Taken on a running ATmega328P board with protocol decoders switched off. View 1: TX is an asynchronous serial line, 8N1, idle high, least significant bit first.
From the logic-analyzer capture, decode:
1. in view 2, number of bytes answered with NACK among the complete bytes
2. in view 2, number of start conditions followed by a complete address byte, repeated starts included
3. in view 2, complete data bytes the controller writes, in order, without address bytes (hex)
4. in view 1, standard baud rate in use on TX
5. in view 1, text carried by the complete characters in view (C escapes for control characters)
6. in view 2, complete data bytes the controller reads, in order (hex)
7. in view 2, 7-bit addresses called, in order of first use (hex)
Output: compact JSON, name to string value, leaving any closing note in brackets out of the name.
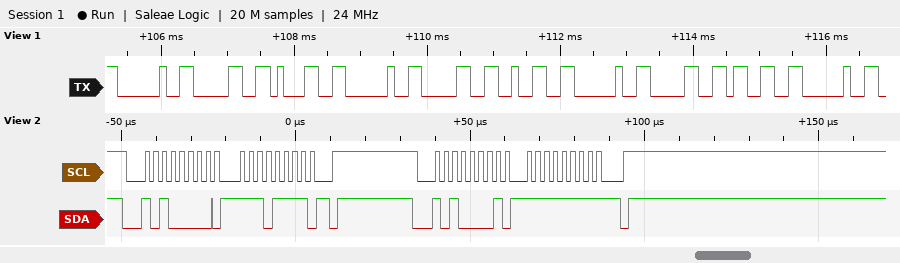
{"in view 2, number of bytes answered with NACK among the complete bytes": "1", "in view 2, number of start conditions followed by a complete address byte, repeated starts included": "2", "in view 2, complete data bytes the controller writes, in order, without address bytes": "EF", "in view 1, standard baud rate in use on TX": "9600 baud", "in view 1, text carried by the complete characters in view": "\" 01 02 03 \"", "in view 2, complete data bytes the controller reads, in order": "FF", "in view 2, 7-bit addresses called, in order of first use": "0x50"}
